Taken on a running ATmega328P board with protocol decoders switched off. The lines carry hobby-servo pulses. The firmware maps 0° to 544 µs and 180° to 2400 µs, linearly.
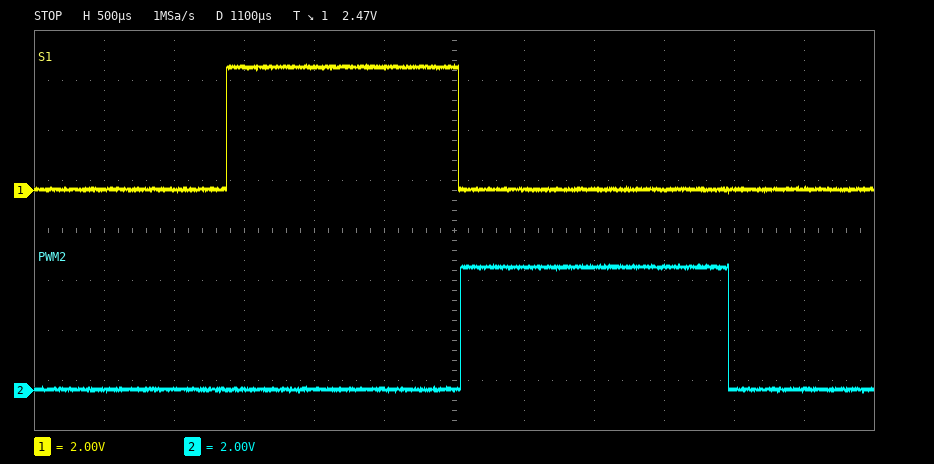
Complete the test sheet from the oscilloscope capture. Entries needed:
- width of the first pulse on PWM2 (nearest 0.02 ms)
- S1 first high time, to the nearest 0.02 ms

1.92 ms
1.66 ms
